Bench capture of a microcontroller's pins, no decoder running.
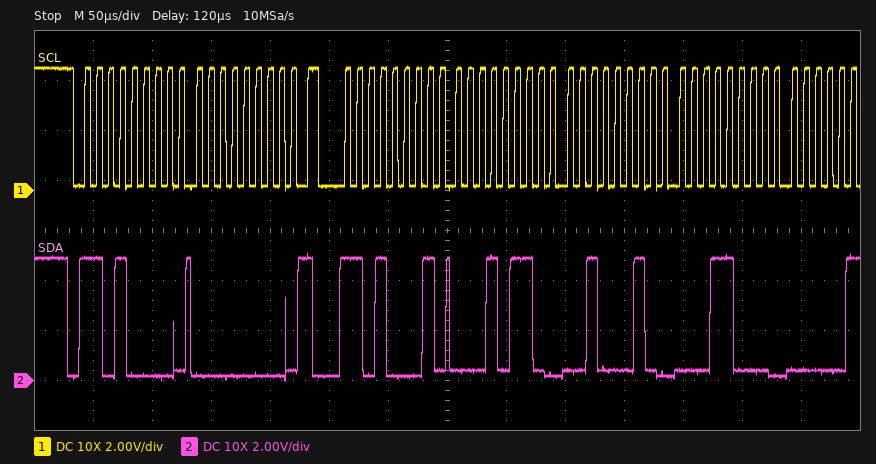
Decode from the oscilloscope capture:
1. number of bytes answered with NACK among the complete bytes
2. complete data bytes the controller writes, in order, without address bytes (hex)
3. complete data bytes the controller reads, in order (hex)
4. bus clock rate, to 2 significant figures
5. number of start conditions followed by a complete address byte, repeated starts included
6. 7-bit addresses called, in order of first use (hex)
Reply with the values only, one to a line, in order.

0
00
16 22 18
100 kHz
2
0x68
